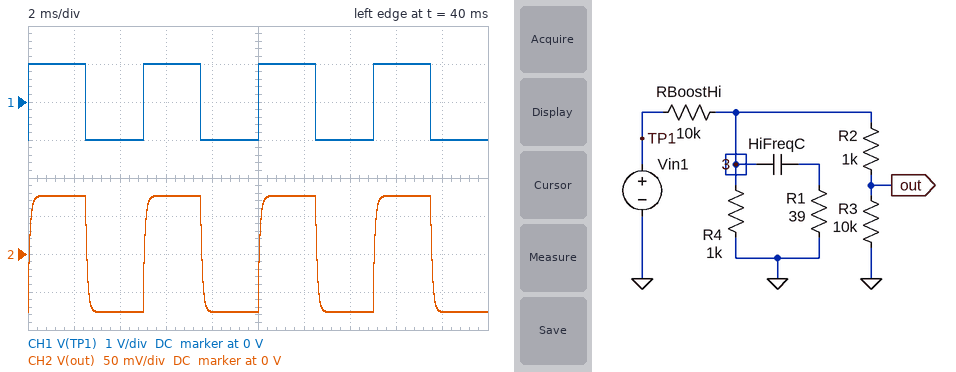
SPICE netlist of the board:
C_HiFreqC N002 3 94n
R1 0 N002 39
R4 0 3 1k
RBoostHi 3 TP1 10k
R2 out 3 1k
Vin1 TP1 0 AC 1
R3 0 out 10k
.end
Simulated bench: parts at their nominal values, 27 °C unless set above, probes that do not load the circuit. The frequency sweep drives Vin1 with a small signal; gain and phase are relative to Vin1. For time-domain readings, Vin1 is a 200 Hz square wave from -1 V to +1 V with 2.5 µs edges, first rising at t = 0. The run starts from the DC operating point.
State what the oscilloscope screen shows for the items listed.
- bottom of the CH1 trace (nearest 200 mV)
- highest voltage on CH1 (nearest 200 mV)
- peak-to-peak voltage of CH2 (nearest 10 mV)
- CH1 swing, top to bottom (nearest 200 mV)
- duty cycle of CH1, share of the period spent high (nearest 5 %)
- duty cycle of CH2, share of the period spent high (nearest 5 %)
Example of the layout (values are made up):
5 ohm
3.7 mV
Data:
-1.0 V
1.0 V
150 mV
2.0 V
50 %
50 %
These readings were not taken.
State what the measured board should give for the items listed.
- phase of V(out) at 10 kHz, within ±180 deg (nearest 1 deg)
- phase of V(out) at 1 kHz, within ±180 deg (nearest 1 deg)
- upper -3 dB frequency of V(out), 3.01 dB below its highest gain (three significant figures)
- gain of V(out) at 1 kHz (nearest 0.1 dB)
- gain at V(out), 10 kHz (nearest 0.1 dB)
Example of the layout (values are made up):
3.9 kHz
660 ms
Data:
-66 deg
-26 deg
1.93 kHz
-23.4 dB
-36.6 dB
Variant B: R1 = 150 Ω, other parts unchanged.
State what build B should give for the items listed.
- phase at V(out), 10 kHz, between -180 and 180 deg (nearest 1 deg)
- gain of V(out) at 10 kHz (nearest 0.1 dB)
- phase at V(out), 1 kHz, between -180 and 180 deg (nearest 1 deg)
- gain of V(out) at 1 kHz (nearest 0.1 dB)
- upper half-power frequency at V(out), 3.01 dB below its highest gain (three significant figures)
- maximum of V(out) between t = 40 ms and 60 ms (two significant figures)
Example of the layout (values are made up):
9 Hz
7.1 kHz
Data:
-39 deg
-35.3 dB
-25 deg
-23.6 dB
1.75 kHz
76 mV
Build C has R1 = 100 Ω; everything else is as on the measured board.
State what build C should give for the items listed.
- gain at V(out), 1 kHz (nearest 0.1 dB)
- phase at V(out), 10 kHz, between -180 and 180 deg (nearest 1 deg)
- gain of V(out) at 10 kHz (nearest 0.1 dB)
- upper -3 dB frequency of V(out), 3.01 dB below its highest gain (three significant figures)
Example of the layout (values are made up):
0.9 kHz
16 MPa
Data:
-23.5 dB
-49 deg
-36.1 dB
1.82 kHz
